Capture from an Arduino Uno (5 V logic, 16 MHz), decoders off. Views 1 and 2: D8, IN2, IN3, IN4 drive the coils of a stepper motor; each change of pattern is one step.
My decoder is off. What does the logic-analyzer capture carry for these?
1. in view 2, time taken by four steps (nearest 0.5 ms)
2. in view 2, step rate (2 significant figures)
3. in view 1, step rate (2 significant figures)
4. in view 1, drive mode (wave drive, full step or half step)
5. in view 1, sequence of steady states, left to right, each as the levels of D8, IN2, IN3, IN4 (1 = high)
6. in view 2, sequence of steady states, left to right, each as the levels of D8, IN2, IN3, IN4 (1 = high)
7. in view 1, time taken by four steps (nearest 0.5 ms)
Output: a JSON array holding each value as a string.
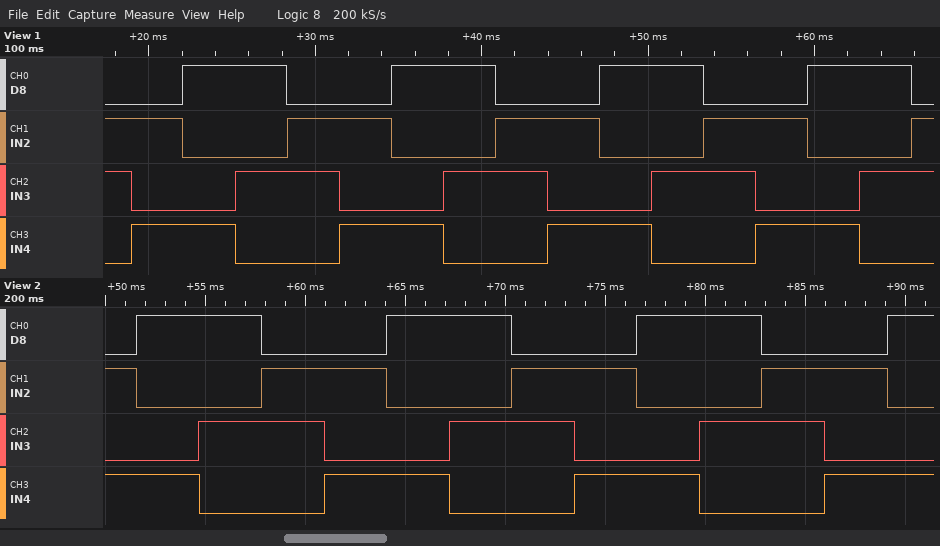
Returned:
["12.5 ms", "320 steps/s", "320 steps/s", "full step", "0110 0101 1001 1010 0110 0101 1001 1010 0110 0101 1001 1010 0110 0101 1001 1010 0110", "0101 1001 1010 0110 0101 1001 1010 0110 0101 1001 1010 0110 0101 1001", "12.5 ms"]
